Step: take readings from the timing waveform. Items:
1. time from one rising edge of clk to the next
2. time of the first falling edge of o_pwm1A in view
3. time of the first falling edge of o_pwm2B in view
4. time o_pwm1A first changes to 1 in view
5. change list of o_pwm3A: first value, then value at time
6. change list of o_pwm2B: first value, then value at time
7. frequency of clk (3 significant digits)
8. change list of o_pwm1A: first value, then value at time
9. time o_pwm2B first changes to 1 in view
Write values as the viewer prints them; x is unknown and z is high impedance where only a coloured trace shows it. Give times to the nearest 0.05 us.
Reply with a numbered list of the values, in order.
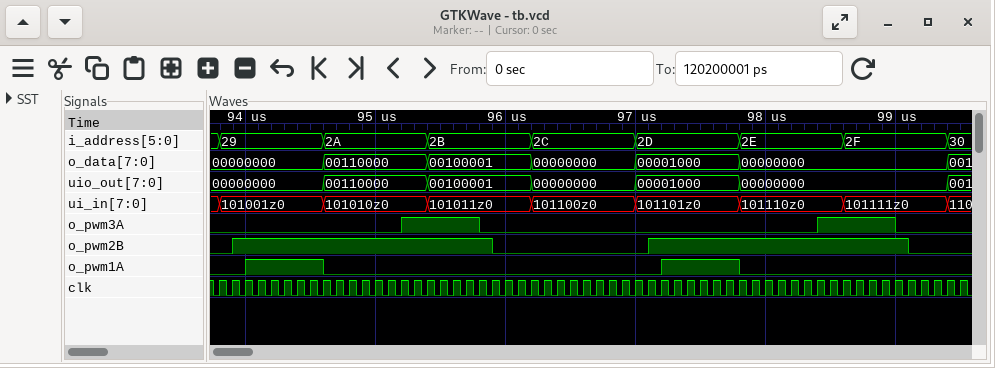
1. 0.1 us
2. 94.6 us
3. 95.9 us
4. 94 us
5. 0, 1 at 95.2 us, 0 at 95.8 us, 1 at 98.4 us, 0 at 99 us
6. 0, 1 at 93.9 us, 0 at 95.9 us, 1 at 97.1 us, 0 at 99.1 us
7. 10.0 MHz
8. 0, 1 at 94 us, 0 at 94.6 us, 1 at 97.2 us, 0 at 97.8 us
9. 93.9 us
